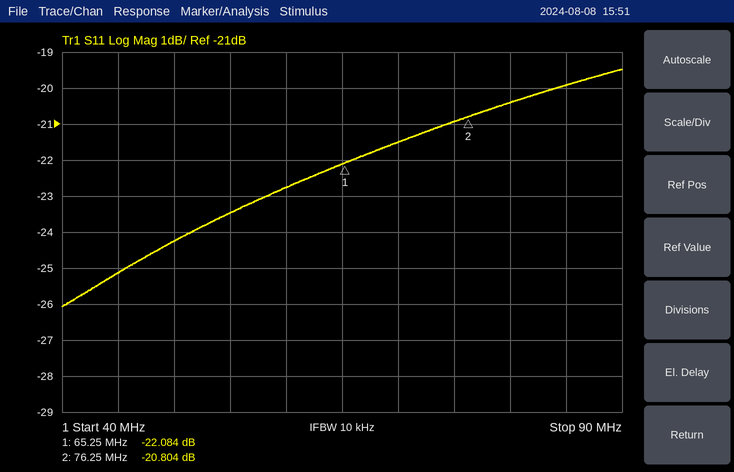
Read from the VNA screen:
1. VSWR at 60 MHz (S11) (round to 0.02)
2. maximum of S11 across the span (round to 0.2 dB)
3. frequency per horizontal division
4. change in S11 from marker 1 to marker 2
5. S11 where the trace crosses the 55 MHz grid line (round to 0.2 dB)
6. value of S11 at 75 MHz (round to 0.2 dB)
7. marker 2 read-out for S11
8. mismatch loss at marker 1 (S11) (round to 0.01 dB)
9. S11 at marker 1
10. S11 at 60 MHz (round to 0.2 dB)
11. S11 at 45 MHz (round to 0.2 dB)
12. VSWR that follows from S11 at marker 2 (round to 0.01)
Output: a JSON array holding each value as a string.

["1.16", "-19.4 dB", "5 MHz", "1.280 dB", "-23.4 dB", "-21.0 dB", "-20.804 dB", "0.03 dB", "-22.084 dB", "-22.8 dB", "-25.2 dB", "1.20"]
